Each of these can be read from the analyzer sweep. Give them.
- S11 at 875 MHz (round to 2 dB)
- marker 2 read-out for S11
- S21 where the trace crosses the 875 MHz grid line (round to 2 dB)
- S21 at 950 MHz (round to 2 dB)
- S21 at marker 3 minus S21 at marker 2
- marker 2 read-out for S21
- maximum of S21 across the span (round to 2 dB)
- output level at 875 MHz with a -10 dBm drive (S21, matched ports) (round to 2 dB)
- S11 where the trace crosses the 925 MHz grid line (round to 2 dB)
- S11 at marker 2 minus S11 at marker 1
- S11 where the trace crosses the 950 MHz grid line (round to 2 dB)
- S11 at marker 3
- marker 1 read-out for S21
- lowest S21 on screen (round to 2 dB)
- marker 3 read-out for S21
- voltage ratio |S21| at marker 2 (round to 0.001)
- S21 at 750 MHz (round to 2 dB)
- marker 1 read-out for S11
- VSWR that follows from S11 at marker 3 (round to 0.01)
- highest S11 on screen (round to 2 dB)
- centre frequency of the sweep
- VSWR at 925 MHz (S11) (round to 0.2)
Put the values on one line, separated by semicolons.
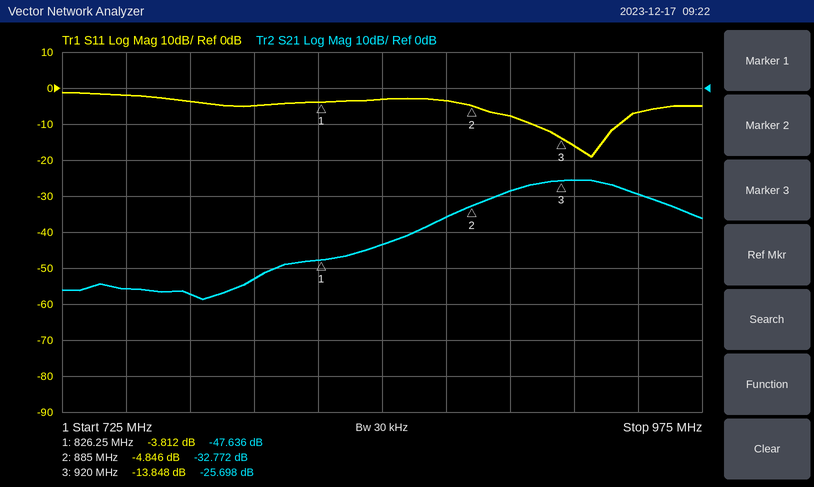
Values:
-4 dB; -4.846 dB; -36 dB; -30 dB; 7.074 dB; -32.772 dB; -26 dB; -46 dBm; -16 dB; -1.034 dB; -6 dB; -13.848 dB; -47.636 dB; -58 dB; -25.698 dB; 0.023; -56 dB; -3.812 dB; 1.51; -2 dB; 850 MHz; 1.4
